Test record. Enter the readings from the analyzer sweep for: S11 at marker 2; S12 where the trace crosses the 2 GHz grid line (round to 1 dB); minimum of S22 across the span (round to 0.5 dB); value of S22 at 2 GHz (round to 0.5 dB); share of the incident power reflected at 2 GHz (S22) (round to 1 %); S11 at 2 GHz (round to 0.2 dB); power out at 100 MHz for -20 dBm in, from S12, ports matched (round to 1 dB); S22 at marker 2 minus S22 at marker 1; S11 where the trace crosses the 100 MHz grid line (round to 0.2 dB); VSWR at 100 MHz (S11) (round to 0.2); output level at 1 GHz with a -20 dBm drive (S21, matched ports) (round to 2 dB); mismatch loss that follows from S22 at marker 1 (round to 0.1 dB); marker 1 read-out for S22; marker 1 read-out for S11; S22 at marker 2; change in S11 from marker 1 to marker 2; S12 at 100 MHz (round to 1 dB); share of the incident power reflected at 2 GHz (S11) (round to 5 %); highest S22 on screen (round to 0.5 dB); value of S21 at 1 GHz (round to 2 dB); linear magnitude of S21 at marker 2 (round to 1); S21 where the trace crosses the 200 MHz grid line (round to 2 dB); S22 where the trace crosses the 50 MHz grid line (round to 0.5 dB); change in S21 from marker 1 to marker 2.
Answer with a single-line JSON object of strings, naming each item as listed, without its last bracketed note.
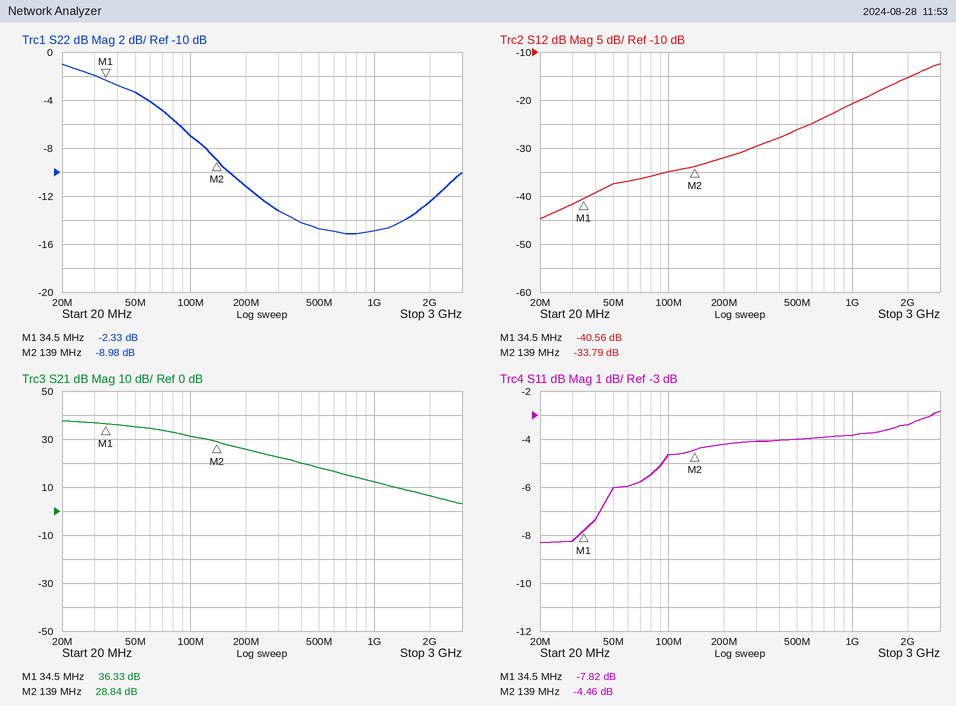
{"S11 at marker 2": "-4.46 dB", "S12 where the trace crosses the 2 GHz grid line": "-15 dB", "minimum of S22 across the span": "-15.0 dB", "value of S22 at 2 GHz": "-12.5 dB", "share of the incident power reflected at 2 GHz (S22)": "6 %", "S11 at 2 GHz": "-3.4 dB", "power out at 100 MHz for -20 dBm in, from S12, ports matched": "-55 dBm", "S22 at marker 2 minus S22 at marker 1": "-6.65 dB", "S11 where the trace crosses the 100 MHz grid line": "-4.6 dB", "VSWR at 100 MHz (S11)": "3.8", "output level at 1 GHz with a -20 dBm drive (S21, matched ports)": "-8 dBm", "mismatch loss that follows from S22 at marker 1": "3.8 dB", "marker 1 read-out for S22": "-2.33 dB", "marker 1 read-out for S11": "-7.82 dB", "S22 at marker 2": "-8.98 dB", "change in S11 from marker 1 to marker 2": "3.36 dB", "S12 at 100 MHz": "-35 dB", "share of the incident power reflected at 2 GHz (S11)": "45 %", "highest S22 on screen": "-1.0 dB", "value of S21 at 1 GHz": "12 dB", "linear magnitude of S21 at marker 2": "28", "S21 where the trace crosses the 200 MHz grid line": "26 dB", "S22 where the trace crosses the 50 MHz grid line": "-3.5 dB", "change in S21 from marker 1 to marker 2": "-7.49 dB"}
